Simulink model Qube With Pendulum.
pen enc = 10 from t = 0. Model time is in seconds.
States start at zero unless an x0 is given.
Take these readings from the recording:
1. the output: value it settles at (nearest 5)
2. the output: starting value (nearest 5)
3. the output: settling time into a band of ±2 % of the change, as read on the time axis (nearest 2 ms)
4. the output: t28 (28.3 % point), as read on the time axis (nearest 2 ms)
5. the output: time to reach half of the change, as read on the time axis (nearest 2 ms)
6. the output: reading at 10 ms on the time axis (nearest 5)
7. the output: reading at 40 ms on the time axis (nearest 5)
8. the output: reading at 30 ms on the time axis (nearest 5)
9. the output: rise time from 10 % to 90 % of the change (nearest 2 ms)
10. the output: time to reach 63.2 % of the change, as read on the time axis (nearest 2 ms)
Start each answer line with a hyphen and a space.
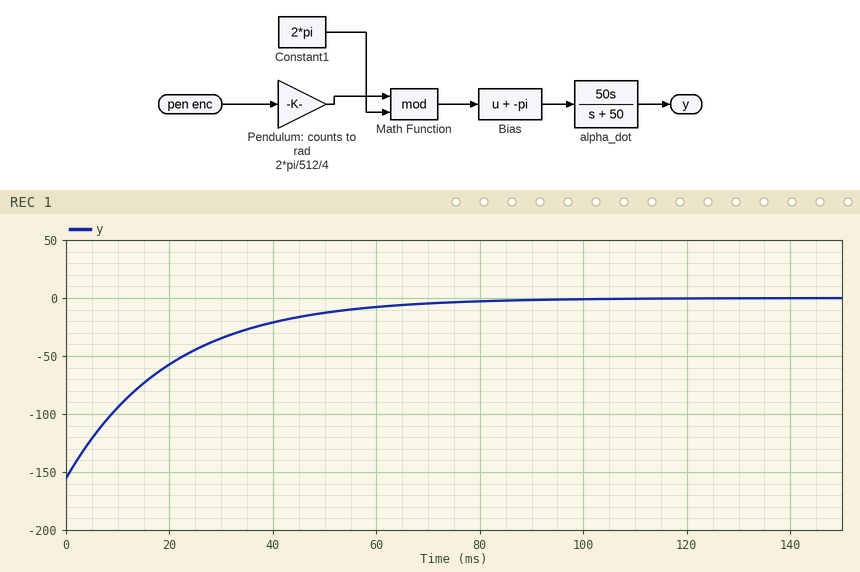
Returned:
- 0
- -155
- 78 ms
- 6 ms
- 14 ms
- -95
- -20
- -35
- 44 ms
- 20 ms
